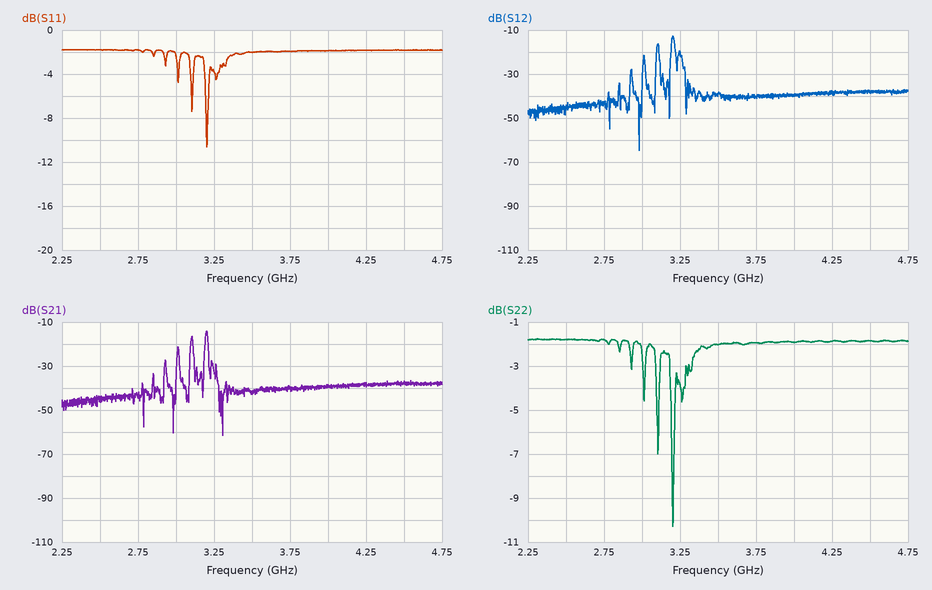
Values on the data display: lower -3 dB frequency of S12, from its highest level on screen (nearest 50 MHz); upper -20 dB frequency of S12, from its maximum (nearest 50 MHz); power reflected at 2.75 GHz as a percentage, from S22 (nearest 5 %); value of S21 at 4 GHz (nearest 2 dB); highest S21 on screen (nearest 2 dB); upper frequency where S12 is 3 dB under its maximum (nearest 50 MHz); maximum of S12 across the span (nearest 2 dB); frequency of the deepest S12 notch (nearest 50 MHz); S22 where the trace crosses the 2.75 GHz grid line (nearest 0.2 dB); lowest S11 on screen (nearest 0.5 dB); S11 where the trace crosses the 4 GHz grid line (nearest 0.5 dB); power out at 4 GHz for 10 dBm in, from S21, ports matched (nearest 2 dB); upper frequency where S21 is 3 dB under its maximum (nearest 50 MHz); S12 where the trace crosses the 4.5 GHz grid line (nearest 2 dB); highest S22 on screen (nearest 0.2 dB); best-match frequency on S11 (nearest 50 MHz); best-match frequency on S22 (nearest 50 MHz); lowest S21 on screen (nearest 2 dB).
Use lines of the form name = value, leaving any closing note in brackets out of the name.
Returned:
lower -3 dB frequency of S12, from its highest level on screen = 3.20 GHz
upper -20 dB frequency of S12, from its maximum = 3.30 GHz
power reflected at 2.75 GHz as a percentage, from S22 = 65 %
value of S21 at 4 GHz = -38 dB
highest S21 on screen = -14 dB
upper frequency where S12 is 3 dB under its maximum = 3.20 GHz
maximum of S12 across the span = -12 dB
frequency of the deepest S12 notch = 3.00 GHz
S22 where the trace crosses the 2.75 GHz grid line = -1.8 dB
lowest S11 on screen = -10.5 dB
S11 where the trace crosses the 4 GHz grid line = -2.0 dB
power out at 4 GHz for 10 dBm in, from S21, ports matched = -28 dBm
upper frequency where S21 is 3 dB under its maximum = 3.20 GHz
S12 where the trace crosses the 4.5 GHz grid line = -38 dB
highest S22 on screen = -1.8 dB
best-match frequency on S11 = 3.20 GHz
best-match frequency on S22 = 3.20 GHz
lowest S21 on screen = -62 dB
